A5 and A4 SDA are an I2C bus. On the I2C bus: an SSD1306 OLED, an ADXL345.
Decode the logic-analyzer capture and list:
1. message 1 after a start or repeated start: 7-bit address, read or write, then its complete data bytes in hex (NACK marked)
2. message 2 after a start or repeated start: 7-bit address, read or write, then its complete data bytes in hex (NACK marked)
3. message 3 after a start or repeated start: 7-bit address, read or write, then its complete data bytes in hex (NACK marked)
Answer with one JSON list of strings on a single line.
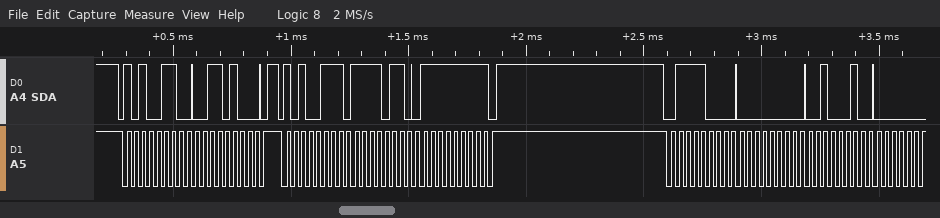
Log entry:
["0x53 write: 34", "0x53 read: F6 FF NACK", "0x3C write: 00 22"]
